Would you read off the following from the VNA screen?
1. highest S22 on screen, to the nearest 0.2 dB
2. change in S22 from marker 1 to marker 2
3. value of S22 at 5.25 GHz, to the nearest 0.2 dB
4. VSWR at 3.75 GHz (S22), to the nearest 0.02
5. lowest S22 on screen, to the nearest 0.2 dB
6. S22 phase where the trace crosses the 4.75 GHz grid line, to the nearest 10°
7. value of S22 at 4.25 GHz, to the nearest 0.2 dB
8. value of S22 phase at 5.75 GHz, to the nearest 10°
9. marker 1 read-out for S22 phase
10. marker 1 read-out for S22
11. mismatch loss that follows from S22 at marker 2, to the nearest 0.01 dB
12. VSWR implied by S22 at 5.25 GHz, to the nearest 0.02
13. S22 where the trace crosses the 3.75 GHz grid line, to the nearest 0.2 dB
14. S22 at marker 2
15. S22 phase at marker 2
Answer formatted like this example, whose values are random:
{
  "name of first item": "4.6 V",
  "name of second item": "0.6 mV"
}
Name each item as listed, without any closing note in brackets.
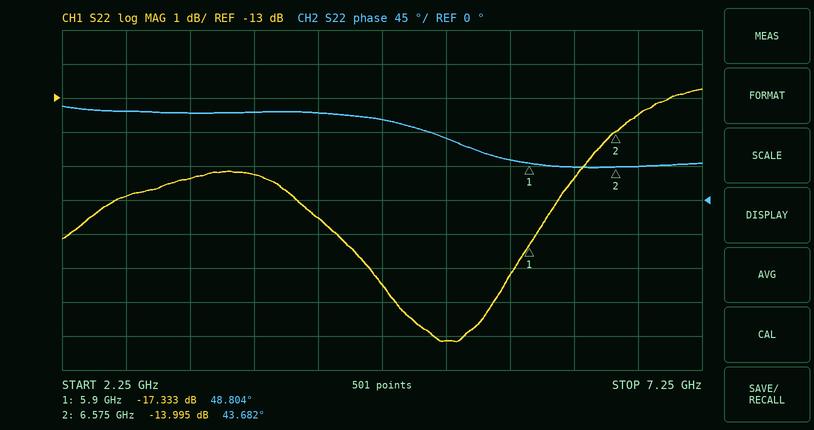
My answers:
{
  "highest S22 on screen, to the nearest 0.2 dB": "-12.8 dB",
  "change in S22 from marker 1 to marker 2": "3.338 dB",
  "value of S22 at 5.25 GHz, to the nearest 0.2 dB": "-20.2 dB",
  "VSWR at 3.75 GHz (S22), to the nearest 0.02": "1.42",
  "lowest S22 on screen, to the nearest 0.2 dB": "-20.2 dB",
  "S22 phase where the trace crosses the 4.75 GHz grid line, to the nearest 10°": "110°",
  "value of S22 at 4.25 GHz, to the nearest 0.2 dB": "-16.6 dB",
  "value of S22 phase at 5.75 GHz, to the nearest 10°": "50°",
  "marker 1 read-out for S22 phase": "48.804°",
  "marker 1 read-out for S22": "-17.333 dB",
  "mismatch loss that follows from S22 at marker 2, to the nearest 0.01 dB": "0.18 dB",
  "VSWR implied by S22 at 5.25 GHz, to the nearest 0.02": "1.22",
  "S22 where the trace crosses the 3.75 GHz grid line, to the nearest 0.2 dB": "-15.2 dB",
  "S22 at marker 2": "-13.995 dB",
  "S22 phase at marker 2": "43.682°"
}
